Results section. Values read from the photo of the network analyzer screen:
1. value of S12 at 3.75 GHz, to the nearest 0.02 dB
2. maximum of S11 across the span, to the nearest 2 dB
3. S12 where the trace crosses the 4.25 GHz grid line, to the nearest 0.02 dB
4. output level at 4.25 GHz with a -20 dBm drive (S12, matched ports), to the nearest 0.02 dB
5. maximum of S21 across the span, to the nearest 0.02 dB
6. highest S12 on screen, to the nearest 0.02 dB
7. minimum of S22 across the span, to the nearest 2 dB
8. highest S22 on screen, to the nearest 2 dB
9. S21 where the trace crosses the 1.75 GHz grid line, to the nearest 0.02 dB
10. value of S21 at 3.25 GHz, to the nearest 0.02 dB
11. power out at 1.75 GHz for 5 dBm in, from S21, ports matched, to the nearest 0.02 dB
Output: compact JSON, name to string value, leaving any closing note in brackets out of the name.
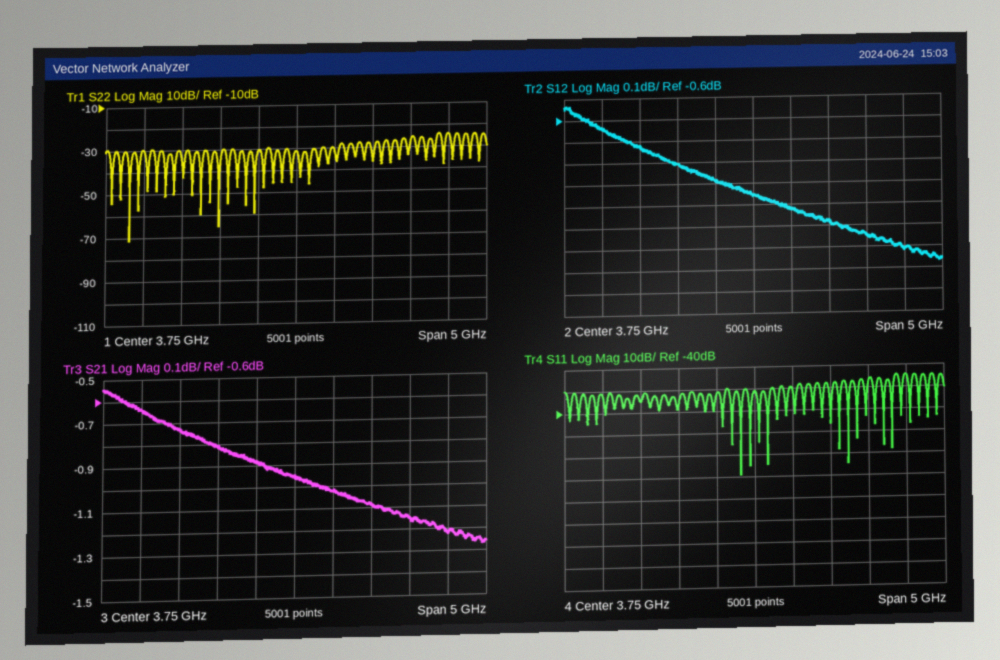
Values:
{"value of S12 at 3.75 GHz, to the nearest 0.02 dB": "-0.96 dB", "maximum of S11 across the span, to the nearest 2 dB": "-24 dB", "S12 where the trace crosses the 4.25 GHz grid line, to the nearest 0.02 dB": "-1.02 dB", "output level at 4.25 GHz with a -20 dBm drive (S12, matched ports), to the nearest 0.02 dB": "-21.02 dBm", "maximum of S21 across the span, to the nearest 0.02 dB": "-0.54 dB", "highest S12 on screen, to the nearest 0.02 dB": "-0.54 dB", "minimum of S22 across the span, to the nearest 2 dB": "-72 dB", "highest S22 on screen, to the nearest 2 dB": "-24 dB", "S21 where the trace crosses the 1.75 GHz grid line, to the nearest 0.02 dB": "-0.64 dB", "value of S21 at 3.25 GHz, to the nearest 0.02 dB": "-0.88 dB", "power out at 1.75 GHz for 5 dBm in, from S21, ports matched, to the nearest 0.02 dB": "4.36 dBm"}
